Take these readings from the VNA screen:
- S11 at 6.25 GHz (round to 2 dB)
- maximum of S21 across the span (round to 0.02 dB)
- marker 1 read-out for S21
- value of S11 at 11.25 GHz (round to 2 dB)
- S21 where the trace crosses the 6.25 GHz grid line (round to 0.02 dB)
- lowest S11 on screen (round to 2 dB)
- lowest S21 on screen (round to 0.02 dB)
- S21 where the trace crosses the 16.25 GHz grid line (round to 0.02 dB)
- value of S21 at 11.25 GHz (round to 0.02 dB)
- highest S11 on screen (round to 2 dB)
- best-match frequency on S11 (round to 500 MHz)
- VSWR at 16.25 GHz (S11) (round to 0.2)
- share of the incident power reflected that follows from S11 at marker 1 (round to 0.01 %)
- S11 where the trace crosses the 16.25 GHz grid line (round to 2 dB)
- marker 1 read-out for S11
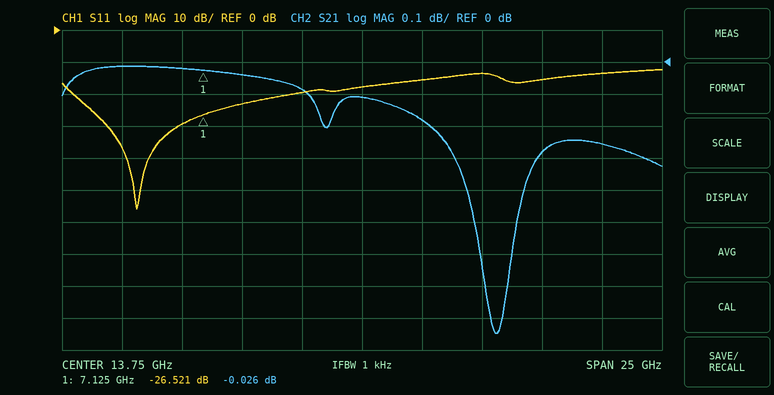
-30 dB
-0.02 dB
-0.026 dB
-20 dB
-0.02 dB
-56 dB
-0.84 dB
-0.18 dB
-0.08 dB
-12 dB
4.5 GHz
1.4
0.22 %
-16 dB
-26.521 dB
